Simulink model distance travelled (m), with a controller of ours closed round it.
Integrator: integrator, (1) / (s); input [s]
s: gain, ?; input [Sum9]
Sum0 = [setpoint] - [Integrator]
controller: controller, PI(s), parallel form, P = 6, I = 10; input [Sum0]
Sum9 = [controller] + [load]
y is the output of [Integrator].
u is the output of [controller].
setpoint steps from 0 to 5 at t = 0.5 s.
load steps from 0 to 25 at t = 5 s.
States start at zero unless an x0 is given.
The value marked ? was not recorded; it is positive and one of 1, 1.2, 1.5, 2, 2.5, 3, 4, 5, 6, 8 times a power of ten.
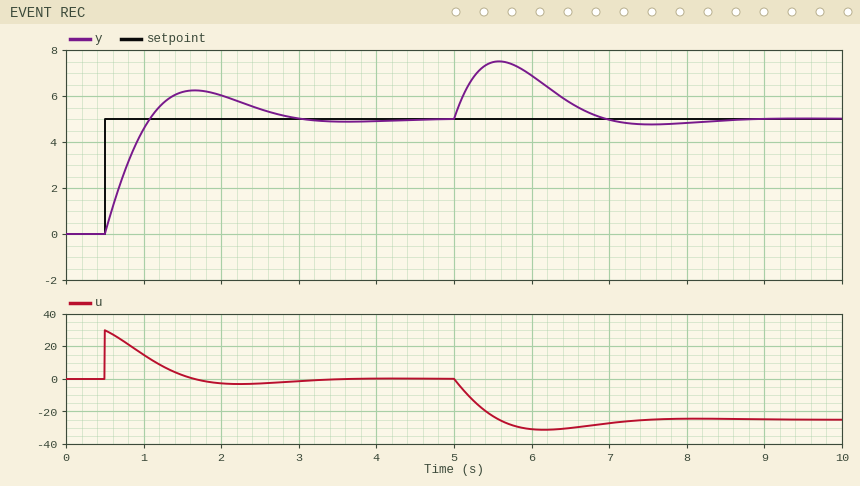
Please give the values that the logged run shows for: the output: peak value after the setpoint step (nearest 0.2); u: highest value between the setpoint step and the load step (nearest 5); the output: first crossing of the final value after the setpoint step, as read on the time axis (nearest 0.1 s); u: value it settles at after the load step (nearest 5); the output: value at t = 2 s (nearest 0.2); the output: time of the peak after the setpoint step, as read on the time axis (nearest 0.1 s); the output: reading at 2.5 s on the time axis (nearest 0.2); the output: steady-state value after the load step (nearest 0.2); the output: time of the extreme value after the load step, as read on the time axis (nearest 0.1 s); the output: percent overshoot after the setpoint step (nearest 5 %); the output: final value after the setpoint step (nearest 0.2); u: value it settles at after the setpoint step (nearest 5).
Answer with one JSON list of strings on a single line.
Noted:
["6.2", "30", "1.1 s", "-25", "6.0", "1.7 s", "5.4", "5.0", "5.6 s", "25 %", "5.0", "0"]
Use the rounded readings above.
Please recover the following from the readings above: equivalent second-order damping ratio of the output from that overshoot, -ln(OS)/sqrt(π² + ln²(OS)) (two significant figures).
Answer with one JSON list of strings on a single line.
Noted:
["0.40"]
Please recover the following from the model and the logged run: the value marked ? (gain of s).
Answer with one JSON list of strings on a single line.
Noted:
["0.4"]
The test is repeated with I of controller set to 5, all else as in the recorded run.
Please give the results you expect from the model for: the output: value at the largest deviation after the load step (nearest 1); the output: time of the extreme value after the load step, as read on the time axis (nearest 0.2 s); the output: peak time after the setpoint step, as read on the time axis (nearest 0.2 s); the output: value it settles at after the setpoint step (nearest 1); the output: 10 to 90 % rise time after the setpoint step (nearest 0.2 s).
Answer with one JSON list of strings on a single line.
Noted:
["8", "5.8 s", "2.0 s", "5", "0.6 s"]
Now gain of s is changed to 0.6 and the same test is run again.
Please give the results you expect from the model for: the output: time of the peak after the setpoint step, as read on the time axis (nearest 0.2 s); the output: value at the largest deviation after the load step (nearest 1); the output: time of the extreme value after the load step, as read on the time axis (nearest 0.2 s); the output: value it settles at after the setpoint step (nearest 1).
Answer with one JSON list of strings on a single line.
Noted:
["1.4 s", "8", "5.4 s", "5"]
